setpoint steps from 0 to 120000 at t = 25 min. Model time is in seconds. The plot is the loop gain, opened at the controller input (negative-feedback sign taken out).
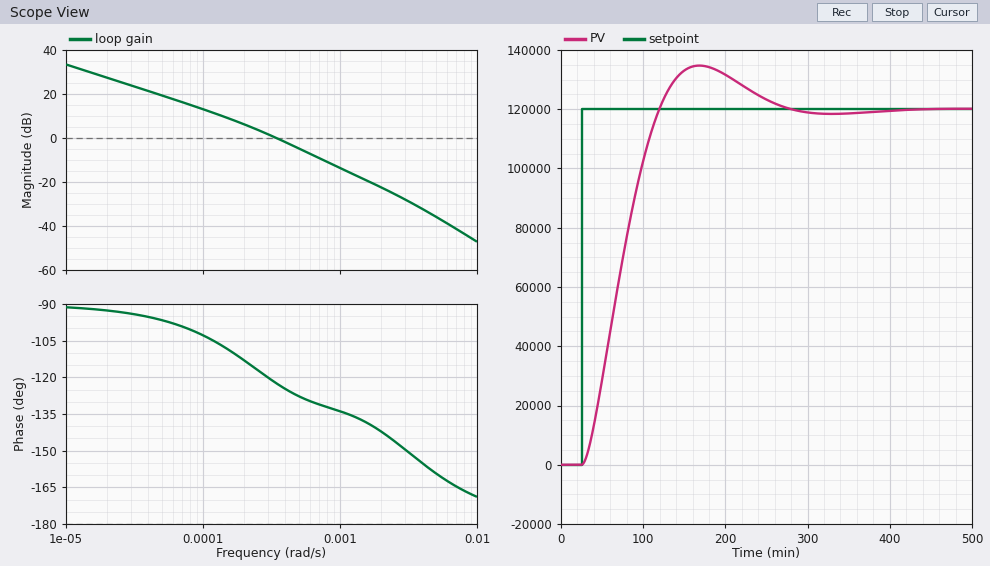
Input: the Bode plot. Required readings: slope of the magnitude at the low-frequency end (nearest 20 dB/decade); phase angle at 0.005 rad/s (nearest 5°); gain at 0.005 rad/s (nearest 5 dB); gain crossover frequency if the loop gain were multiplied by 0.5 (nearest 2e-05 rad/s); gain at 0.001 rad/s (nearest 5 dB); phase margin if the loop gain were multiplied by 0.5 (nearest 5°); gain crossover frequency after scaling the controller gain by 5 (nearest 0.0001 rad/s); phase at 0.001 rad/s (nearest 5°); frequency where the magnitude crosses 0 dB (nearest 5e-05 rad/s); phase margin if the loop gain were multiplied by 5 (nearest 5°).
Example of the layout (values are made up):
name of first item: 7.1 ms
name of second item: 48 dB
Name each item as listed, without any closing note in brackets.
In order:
slope of the magnitude at the low-frequency end: -20 dB/decade
phase angle at 0.005 rad/s: -160°
gain at 0.005 rad/s: -35 dB
gain crossover frequency if the loop gain were multiplied by 0.5: 0.00020 rad/s
gain at 0.001 rad/s: -15 dB
phase margin if the loop gain were multiplied by 0.5: 65°
gain crossover frequency after scaling the controller gain by 5: 0.0010 rad/s
phase at 0.001 rad/s: -135°
frequency where the magnitude crosses 0 dB: 0.00035 rad/s
phase margin if the loop gain were multiplied by 5: 45°
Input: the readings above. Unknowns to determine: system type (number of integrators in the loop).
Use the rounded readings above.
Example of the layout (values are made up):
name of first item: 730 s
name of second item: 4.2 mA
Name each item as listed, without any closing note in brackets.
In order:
system type: 1
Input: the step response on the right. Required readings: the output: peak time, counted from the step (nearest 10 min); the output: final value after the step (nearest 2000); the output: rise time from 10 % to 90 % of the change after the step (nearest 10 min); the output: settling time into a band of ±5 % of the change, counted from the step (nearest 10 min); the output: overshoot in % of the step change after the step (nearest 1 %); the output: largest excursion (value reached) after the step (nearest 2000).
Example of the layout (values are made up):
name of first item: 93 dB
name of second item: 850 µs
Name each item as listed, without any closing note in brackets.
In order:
the output: peak time, counted from the step: 140 min
the output: final value after the step: 120000
the output: rise time from 10 % to 90 % of the change after the step: 70 min
the output: settling time into a band of ±5 % of the change, counted from the step: 210 min
the output: overshoot in % of the step change after the step: 12 %
the output: largest excursion (value reached) after the step: 134000
